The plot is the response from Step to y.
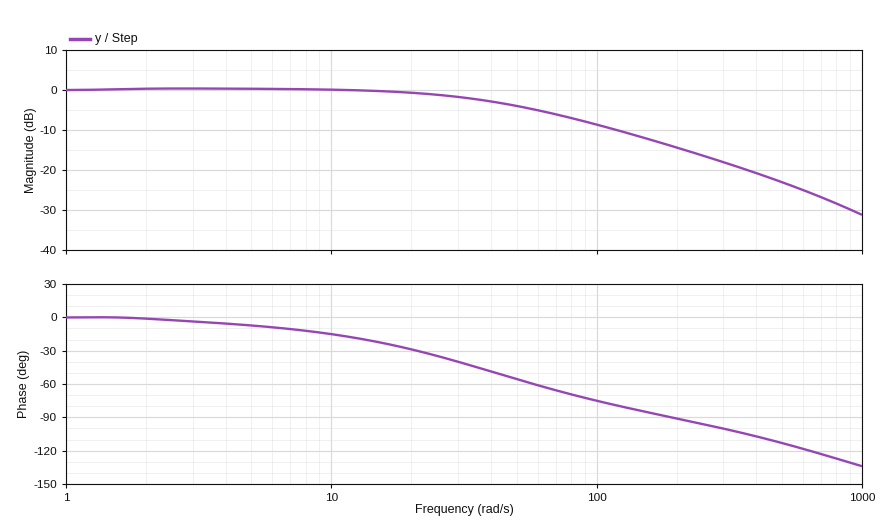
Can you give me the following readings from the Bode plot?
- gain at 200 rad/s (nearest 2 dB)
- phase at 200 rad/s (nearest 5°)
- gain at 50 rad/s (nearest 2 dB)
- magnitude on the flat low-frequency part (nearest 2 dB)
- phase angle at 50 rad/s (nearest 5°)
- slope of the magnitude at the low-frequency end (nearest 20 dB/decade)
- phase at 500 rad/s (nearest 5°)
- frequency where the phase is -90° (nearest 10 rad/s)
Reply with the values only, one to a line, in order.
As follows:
-14 dB
-90°
-4 dB
0 dB
-55°
0 dB/decade
-115°
190 rad/s
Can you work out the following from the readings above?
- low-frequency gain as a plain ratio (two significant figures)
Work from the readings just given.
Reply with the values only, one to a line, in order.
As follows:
1.0
